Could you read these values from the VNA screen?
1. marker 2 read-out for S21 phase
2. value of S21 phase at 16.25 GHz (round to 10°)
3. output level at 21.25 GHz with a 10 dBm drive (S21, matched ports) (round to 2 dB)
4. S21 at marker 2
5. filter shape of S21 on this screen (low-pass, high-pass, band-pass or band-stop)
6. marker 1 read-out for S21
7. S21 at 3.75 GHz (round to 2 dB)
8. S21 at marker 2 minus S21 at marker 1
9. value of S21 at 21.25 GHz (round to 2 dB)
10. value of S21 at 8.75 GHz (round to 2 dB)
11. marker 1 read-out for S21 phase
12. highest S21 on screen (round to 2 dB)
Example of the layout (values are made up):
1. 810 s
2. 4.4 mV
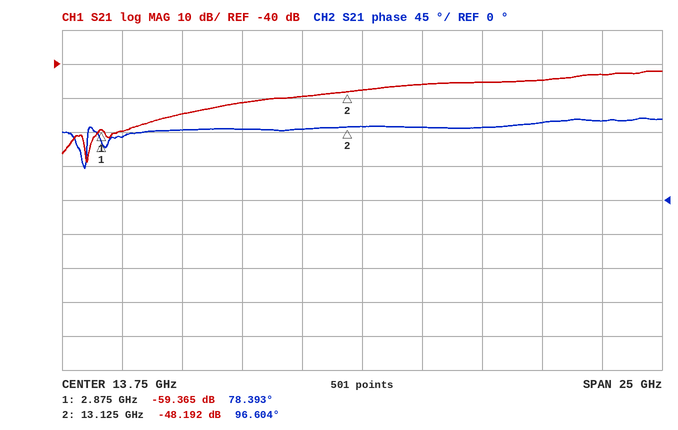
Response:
1. 96.604°
2. 100°
3. -34 dBm
4. -48.192 dB
5. high-pass
6. -59.365 dB
7. -60 dB
8. 11.173 dB
9. -44 dB
10. -52 dB
11. 78.393°
12. -42 dB
